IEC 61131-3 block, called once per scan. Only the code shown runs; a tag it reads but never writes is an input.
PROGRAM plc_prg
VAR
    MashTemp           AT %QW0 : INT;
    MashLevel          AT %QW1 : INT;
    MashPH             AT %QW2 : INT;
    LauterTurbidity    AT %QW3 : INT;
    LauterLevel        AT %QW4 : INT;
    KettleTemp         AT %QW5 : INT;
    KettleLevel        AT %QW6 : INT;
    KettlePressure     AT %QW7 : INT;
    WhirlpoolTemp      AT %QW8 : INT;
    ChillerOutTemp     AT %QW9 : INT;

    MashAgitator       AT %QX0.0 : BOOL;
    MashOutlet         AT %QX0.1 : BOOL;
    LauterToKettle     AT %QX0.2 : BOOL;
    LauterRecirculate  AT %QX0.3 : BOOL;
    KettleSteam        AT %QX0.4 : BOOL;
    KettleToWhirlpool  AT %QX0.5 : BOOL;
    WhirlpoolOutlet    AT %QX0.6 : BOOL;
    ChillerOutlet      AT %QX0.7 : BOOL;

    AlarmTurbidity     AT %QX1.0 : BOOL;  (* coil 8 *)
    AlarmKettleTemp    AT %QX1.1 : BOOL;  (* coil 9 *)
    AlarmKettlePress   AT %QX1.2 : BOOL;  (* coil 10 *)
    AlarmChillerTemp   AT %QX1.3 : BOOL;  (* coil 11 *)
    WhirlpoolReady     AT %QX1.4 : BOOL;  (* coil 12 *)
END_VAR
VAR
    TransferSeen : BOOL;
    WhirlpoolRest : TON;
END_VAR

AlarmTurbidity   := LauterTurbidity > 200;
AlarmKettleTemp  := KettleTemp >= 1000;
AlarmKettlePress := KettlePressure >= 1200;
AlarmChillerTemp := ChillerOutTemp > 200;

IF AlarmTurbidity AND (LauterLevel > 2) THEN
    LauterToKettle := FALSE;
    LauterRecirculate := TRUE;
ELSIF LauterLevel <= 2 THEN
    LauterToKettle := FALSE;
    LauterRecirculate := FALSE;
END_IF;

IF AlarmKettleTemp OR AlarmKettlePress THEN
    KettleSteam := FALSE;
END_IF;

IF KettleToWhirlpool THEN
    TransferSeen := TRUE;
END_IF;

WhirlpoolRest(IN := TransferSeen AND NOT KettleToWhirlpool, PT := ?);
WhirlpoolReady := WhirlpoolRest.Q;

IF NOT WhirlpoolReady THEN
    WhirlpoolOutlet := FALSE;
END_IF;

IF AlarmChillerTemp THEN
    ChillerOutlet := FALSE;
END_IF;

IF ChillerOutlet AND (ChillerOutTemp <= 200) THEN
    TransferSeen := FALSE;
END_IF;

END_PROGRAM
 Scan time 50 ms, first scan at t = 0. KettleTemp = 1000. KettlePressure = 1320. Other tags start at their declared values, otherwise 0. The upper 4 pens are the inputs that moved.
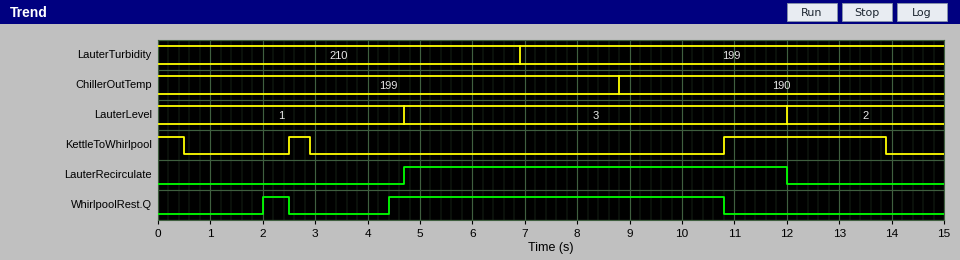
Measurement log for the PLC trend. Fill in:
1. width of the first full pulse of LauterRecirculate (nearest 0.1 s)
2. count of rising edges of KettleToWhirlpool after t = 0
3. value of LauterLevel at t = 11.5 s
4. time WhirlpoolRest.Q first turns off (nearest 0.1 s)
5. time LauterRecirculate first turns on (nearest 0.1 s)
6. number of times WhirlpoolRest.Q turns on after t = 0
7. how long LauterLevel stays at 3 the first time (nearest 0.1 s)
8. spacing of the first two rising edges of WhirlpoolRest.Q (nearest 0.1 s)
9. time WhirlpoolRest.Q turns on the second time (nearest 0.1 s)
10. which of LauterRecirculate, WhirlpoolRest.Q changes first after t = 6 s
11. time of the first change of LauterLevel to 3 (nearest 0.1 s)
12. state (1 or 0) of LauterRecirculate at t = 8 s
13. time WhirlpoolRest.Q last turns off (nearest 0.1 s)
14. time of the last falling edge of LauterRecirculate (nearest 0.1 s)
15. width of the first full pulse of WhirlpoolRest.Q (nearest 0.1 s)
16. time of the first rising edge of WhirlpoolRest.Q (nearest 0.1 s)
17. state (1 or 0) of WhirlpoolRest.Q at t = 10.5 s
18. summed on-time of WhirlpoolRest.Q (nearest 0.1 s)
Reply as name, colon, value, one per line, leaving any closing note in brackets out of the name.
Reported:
width of the first full pulse of LauterRecirculate: 7.3 s
count of rising edges of KettleToWhirlpool after t = 0: 2
value of LauterLevel at t = 11.5 s: 3
time WhirlpoolRest.Q first turns off: 2.5 s
time LauterRecirculate first turns on: 4.7 s
number of times WhirlpoolRest.Q turns on after t = 0: 2
how long LauterLevel stays at 3 the first time: 7.3 s
spacing of the first two rising edges of WhirlpoolRest.Q: 2.4 s
time WhirlpoolRest.Q turns on the second time: 4.4 s
which of LauterRecirculate, WhirlpoolRest.Q changes first after t = 6 s: WhirlpoolRest.Q
time of the first change of LauterLevel to 3: 4.7 s
state (1 or 0) of LauterRecirculate at t = 8 s: 1
time WhirlpoolRest.Q last turns off: 10.8 s
time of the last falling edge of LauterRecirculate: 12.0 s
width of the first full pulse of WhirlpoolRest.Q: 0.5 s
time of the first rising edge of WhirlpoolRest.Q: 2.0 s
state (1 or 0) of WhirlpoolRest.Q at t = 10.5 s: 1
summed on-time of WhirlpoolRest.Q: 6.9 s
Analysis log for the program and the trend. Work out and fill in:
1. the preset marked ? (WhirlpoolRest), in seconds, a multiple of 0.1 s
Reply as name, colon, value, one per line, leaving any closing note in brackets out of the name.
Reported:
the preset marked ? (WhirlpoolRest), in seconds, a multiple of 0.1 s: 1.5 s
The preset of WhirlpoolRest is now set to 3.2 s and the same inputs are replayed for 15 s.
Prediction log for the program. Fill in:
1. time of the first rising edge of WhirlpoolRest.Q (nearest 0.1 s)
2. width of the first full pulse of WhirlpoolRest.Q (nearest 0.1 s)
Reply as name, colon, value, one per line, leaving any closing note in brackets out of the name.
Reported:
time of the first rising edge of WhirlpoolRest.Q: 6.1 s
width of the first full pulse of WhirlpoolRest.Q: 4.7 s
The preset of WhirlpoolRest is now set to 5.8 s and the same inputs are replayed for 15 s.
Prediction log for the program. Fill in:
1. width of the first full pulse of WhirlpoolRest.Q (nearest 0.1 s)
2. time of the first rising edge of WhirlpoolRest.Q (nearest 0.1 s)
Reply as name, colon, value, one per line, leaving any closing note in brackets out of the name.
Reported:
width of the first full pulse of WhirlpoolRest.Q: 2.1 s
time of the first rising edge of WhirlpoolRest.Q: 8.7 s
